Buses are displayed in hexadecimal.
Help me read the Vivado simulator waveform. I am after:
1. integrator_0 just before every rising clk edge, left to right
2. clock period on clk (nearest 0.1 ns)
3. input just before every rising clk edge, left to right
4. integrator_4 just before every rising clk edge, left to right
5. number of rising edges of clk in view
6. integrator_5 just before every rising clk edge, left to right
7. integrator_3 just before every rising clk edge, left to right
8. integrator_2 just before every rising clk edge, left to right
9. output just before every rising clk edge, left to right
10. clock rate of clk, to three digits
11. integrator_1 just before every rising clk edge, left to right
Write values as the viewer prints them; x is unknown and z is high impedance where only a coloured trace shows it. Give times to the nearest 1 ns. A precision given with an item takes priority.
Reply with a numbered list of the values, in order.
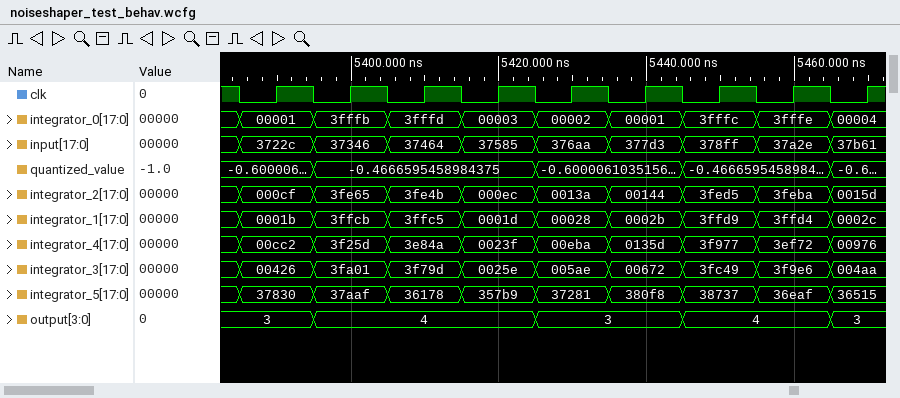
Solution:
1. 00001, 3fffb, 3fffd, 00003, 00002, 00001, 3fffc, 3fffe, 00004
2. 10 ns
3. 3722c, 37346, 37464, 37585, 376aa, 377d3, 378ff, 37a2e, 37b61
4. 00cc2, 3f25d, 3e84a, 0023f, 00eba, 0135d, 3f977, 3ef72, 00976
5. 9
6. 37830, 37aaf, 36178, 357b9, 37281, 380f8, 38737, 36eaf, 36515
7. 00426, 3fa01, 3f79d, 0025e, 005ae, 00672, 3fc49, 3f9e6, 004aa
8. 000cf, 3fe65, 3fe4b, 000ec, 0013a, 00144, 3fed5, 3feba, 0015d
9. 3, 4, 4, 4, 3, 3, 4, 4, 3
10. 100 MHz
11. 0001b, 3ffcb, 3ffc5, 0001d, 00028, 0002b, 3ffd9, 3ffd4, 0002c
